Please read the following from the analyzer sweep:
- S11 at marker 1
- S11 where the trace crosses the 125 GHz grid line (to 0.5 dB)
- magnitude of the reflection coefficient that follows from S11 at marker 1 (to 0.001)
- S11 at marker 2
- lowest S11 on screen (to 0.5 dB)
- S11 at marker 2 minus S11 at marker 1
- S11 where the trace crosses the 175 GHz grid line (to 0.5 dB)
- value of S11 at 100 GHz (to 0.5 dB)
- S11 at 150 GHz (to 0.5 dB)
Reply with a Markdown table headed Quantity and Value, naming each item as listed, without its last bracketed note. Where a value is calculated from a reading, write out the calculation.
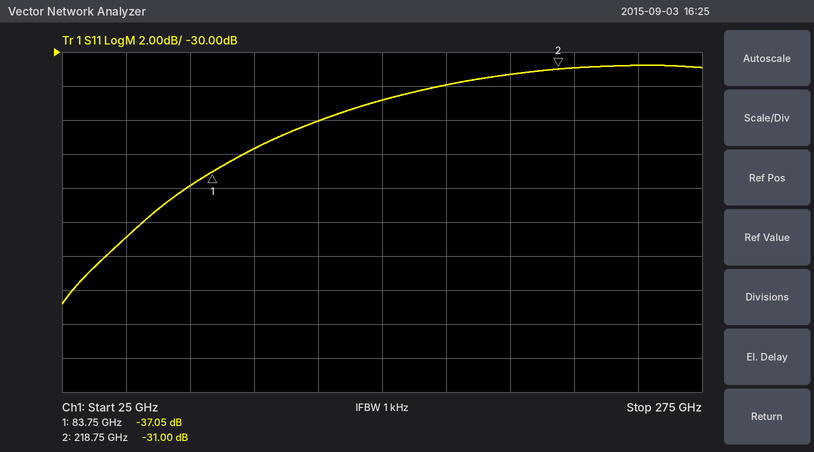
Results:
| Quantity | Value |
|---|---|
| S11 at marker 1 | -37.05 dB |
| S11 where the trace crosses the 125 GHz grid line | -34.0 dB |
| magnitude of the reflection coefficient that follows from S11 at marker 1 | 10^(-37.05/20) ≈ 0.014 |
| S11 at marker 2 | -31.00 dB |
| lowest S11 on screen | -45.0 dB |
| S11 at marker 2 minus S11 at marker 1 | -31 − (-37.05) = 6.05 dB |
| S11 where the trace crosses the 175 GHz grid line | -32.0 dB |
| value of S11 at 100 GHz | -35.5 dB |
| S11 at 150 GHz | -33.0 dB |
